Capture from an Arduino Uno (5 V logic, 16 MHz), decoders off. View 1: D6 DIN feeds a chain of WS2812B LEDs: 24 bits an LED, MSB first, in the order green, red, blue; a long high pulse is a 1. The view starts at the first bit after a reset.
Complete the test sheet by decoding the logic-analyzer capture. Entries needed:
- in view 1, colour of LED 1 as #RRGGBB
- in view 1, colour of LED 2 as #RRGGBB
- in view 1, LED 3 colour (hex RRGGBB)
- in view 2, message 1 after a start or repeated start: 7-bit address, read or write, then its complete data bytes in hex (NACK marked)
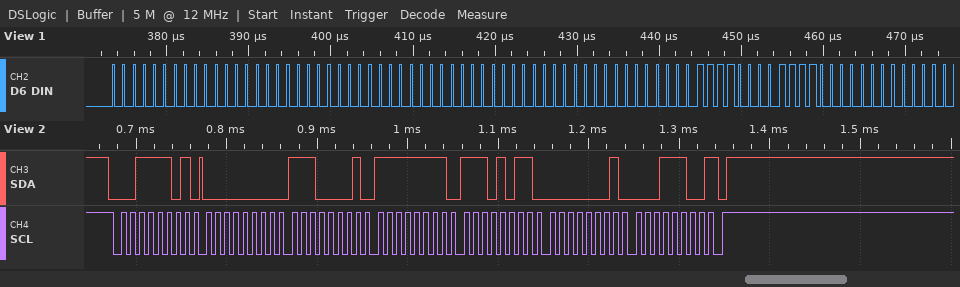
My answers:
#000000
#000000
#780078
0x1E read: 00 E1 FF EB 01 1C NACK
